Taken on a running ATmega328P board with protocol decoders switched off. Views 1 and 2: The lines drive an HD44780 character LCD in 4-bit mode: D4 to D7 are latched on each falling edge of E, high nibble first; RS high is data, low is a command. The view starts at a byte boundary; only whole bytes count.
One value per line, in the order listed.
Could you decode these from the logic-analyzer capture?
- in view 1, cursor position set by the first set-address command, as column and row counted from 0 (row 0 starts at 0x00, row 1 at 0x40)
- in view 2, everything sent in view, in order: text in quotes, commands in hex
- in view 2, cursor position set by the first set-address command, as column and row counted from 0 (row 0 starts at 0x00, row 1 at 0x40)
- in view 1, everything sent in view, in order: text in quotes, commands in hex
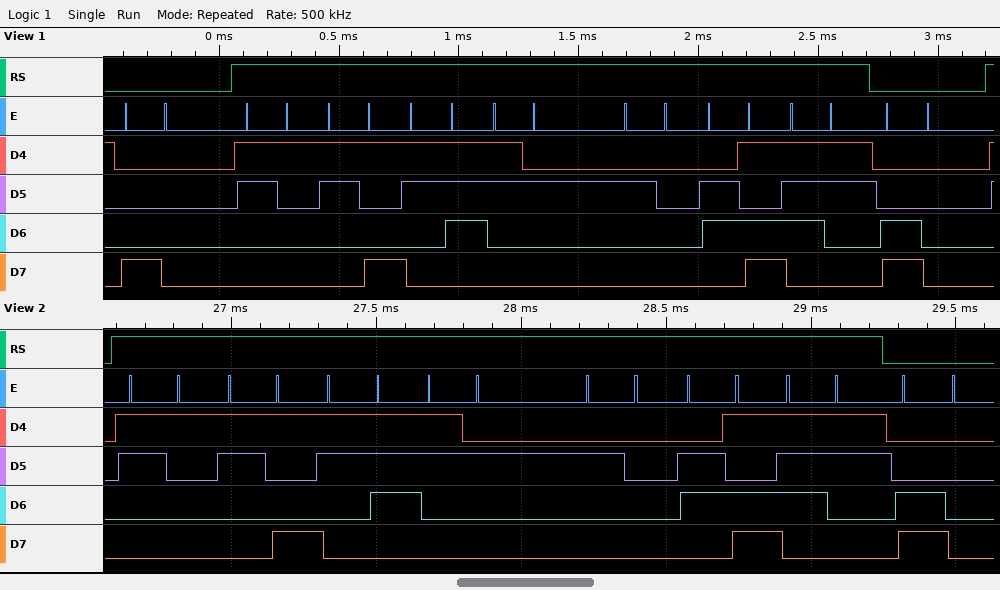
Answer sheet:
column 0, row 0
"1972 ms" 0xC0
column 0, row 1
0x80 "1972 ms" 0xC0
